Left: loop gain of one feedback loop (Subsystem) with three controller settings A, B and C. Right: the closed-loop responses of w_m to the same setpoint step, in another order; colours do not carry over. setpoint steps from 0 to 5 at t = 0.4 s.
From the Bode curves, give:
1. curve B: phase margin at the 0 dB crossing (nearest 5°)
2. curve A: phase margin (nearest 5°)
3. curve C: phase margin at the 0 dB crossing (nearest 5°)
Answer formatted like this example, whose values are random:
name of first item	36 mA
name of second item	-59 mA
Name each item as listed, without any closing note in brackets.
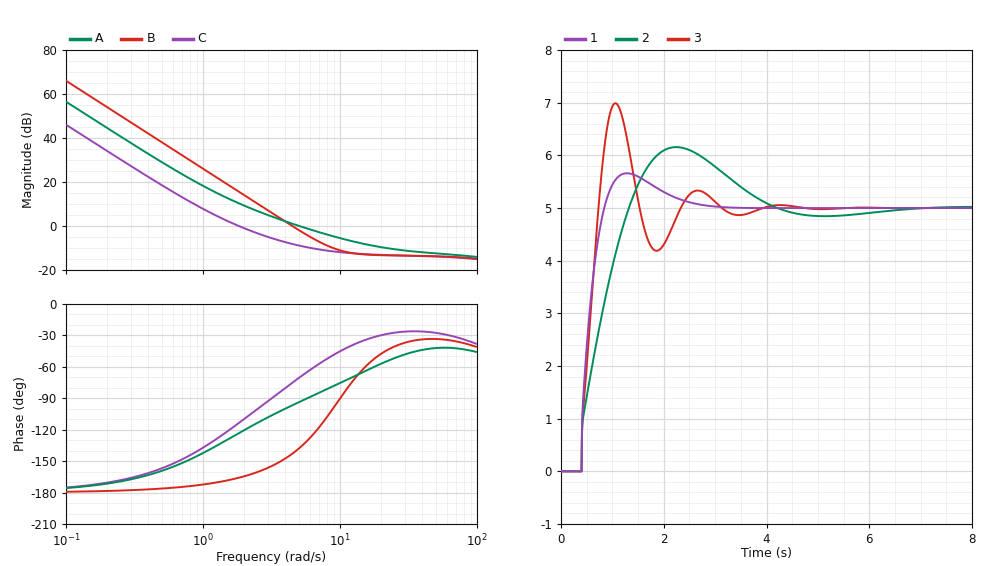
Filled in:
curve B: phase margin at the 0 dB crossing	35°
curve A: phase margin	85°
curve C: phase margin at the 0 dB crossing	65°
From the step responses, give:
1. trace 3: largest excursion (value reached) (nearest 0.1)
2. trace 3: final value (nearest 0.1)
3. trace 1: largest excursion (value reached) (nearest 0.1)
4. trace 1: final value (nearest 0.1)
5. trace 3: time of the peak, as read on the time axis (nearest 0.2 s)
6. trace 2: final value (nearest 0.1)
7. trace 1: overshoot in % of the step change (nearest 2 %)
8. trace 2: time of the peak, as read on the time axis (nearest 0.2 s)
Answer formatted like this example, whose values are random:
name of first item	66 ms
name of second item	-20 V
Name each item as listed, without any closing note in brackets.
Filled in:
trace 3: largest excursion (value reached)	7.0
trace 3: final value	5.0
trace 1: largest excursion (value reached)	5.7
trace 1: final value	5.0
trace 3: time of the peak, as read on the time axis	1.0 s
trace 2: final value	5.0
trace 1: overshoot in % of the step change	14 %
trace 2: time of the peak, as read on the time axis	2.2 s
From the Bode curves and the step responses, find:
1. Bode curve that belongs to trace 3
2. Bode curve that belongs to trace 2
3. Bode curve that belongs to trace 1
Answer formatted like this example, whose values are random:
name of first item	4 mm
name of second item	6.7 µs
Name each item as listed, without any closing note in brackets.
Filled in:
Bode curve that belongs to trace 3	B
Bode curve that belongs to trace 2	C
Bode curve that belongs to trace 1	A
